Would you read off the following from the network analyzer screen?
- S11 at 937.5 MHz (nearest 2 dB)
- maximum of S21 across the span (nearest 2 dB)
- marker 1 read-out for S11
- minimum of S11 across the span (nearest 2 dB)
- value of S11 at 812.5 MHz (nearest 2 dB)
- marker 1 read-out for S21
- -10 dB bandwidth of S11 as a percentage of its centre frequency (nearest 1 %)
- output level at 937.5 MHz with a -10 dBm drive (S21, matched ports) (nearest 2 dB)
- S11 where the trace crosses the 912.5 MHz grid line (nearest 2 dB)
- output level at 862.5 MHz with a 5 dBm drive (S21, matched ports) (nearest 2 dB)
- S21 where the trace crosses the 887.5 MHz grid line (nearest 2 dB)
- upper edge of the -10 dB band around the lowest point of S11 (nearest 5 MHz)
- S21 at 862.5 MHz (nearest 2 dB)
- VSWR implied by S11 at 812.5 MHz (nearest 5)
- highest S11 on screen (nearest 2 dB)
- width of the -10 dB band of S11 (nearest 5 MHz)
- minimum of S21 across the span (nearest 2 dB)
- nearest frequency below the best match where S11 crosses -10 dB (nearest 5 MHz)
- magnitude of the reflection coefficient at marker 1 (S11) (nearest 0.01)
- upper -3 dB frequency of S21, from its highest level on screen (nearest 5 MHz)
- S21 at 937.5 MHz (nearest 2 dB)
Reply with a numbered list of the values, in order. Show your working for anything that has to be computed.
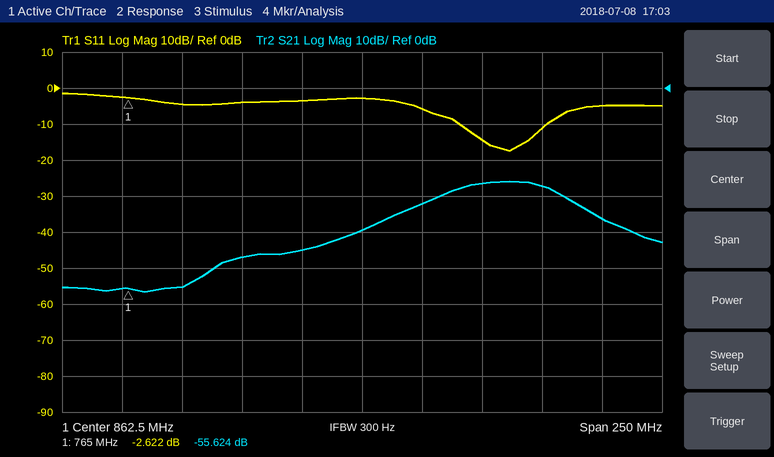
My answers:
1. -12 dB
2. -26 dB
3. -2.622 dB
4. -18 dB
5. -4 dB
6. -55.624 dB
7. 35 MHz / 922.5 MHz ≈ 4 %
8. -10 dBm + (-28 dB) = -38 dBm
9. -14 dB
10. 5 dBm + (-40 dB) = -34 dBm
11. -32 dB
12. 940 MHz
13. -40 dB
14. |Γ| = 10^(-4/20) = 0.6310; VSWR = (1 + 0.6310)/(1 − 0.6310) ≈ 4.42, so 5 to the nearest 5
15. -2 dB
16. 940 MHz − 905 MHz = 35 MHz
17. -56 dB
18. 905 MHz
19. 10^(-2.622/20) ≈ 0.74
20. 945 MHz
21. -28 dB
